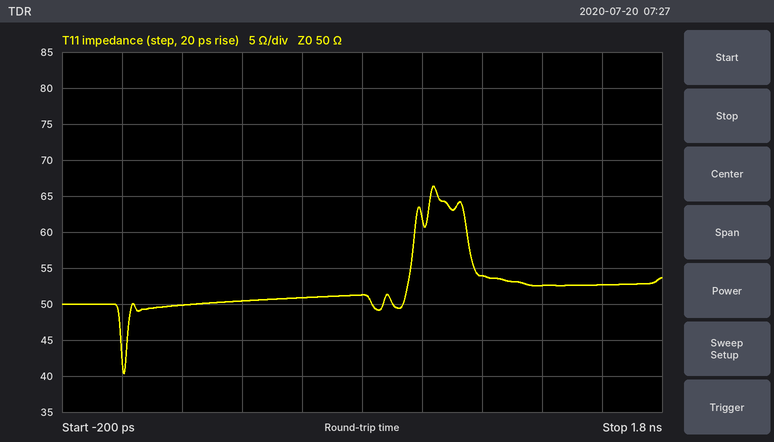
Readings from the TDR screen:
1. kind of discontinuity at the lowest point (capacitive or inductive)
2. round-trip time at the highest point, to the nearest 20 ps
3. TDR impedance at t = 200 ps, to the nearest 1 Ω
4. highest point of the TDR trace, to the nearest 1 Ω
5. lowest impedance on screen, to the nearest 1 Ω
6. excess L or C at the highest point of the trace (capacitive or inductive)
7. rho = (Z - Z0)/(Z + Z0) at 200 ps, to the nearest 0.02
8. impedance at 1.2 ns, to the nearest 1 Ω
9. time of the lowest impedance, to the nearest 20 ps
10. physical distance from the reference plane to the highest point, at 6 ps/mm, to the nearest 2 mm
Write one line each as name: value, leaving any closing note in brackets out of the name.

kind of discontinuity at the lowest point: capacitive
round-trip time at the highest point, to the nearest 20 ps: 1.04 ns
TDR impedance at t = 200 ps, to the nearest 1 Ω: 50 Ω
highest point of the TDR trace, to the nearest 1 Ω: 66 Ω
lowest impedance on screen, to the nearest 1 Ω: 40 Ω
excess L or C at the highest point of the trace: inductive
rho = (Z - Z0)/(Z + Z0) at 200 ps, to the nearest 0.02: 0.00
impedance at 1.2 ns, to the nearest 1 Ω: 54 Ω
time of the lowest impedance, to the nearest 20 ps: 0 ps
physical distance from the reference plane to the highest point, at 6 ps/mm, to the nearest 2 mm: 86 mm
